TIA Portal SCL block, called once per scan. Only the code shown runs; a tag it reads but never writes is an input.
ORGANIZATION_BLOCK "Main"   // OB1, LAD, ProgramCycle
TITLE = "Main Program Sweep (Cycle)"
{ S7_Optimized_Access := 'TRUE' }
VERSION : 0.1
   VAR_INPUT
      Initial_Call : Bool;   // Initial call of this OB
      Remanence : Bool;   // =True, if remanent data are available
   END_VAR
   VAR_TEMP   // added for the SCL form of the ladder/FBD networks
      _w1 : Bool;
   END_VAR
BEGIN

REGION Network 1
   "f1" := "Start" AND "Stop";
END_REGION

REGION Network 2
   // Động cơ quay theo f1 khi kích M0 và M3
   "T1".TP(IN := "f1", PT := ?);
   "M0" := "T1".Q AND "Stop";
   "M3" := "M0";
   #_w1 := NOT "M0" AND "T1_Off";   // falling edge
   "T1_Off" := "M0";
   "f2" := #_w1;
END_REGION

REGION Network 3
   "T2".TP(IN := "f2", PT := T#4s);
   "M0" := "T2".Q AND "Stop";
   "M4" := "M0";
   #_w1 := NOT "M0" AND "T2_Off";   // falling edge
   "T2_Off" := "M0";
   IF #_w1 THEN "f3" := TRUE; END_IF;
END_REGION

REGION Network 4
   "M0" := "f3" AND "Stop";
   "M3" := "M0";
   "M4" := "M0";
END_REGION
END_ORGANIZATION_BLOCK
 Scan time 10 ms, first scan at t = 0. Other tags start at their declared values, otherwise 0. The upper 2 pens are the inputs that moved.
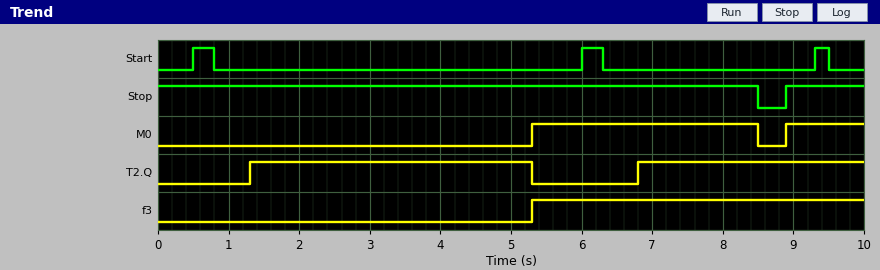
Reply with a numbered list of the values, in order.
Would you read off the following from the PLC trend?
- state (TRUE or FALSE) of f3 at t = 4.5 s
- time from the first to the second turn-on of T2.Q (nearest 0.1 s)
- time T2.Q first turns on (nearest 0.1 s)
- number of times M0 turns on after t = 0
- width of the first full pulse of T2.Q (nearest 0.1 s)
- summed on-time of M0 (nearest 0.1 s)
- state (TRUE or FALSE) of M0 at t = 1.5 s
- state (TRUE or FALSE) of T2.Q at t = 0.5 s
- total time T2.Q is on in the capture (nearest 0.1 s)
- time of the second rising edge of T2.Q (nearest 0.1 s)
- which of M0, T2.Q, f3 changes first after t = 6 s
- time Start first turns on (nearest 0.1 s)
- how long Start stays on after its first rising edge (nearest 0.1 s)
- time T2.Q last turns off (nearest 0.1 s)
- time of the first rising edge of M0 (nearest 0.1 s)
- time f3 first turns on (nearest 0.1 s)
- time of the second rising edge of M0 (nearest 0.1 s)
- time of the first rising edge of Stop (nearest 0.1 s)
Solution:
1. FALSE
2. 5.5 s
3. 1.3 s
4. 2
5. 4.0 s
6. 4.3 s
7. FALSE
8. FALSE
9. 7.2 s
10. 6.8 s
11. T2.Q
12. 0.5 s
13. 0.3 s
14. 5.3 s
15. 5.3 s
16. 5.3 s
17. 8.9 s
18. 8.9 s
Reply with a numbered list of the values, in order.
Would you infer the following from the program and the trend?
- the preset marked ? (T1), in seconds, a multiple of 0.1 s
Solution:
1. 0.8 s
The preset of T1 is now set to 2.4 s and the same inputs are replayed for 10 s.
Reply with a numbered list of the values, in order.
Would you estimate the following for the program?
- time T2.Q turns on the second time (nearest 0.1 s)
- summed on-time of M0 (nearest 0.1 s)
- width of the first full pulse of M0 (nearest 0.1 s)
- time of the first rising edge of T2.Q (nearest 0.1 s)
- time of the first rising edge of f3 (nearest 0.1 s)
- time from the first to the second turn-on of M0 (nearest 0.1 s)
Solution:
1. 8.4 s
2. 2.7 s
3. 1.6 s
4. 2.9 s
5. 6.9 s
6. 2.0 s
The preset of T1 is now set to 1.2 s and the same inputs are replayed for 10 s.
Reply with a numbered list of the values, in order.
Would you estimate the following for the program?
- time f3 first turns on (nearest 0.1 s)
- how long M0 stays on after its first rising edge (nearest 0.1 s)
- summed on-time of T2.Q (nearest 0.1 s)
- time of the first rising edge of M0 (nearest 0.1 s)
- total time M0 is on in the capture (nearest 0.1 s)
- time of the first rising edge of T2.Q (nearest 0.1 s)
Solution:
1. 5.7 s
2. 2.8 s
3. 6.8 s
4. 5.7 s
5. 3.9 s
6. 1.7 s
